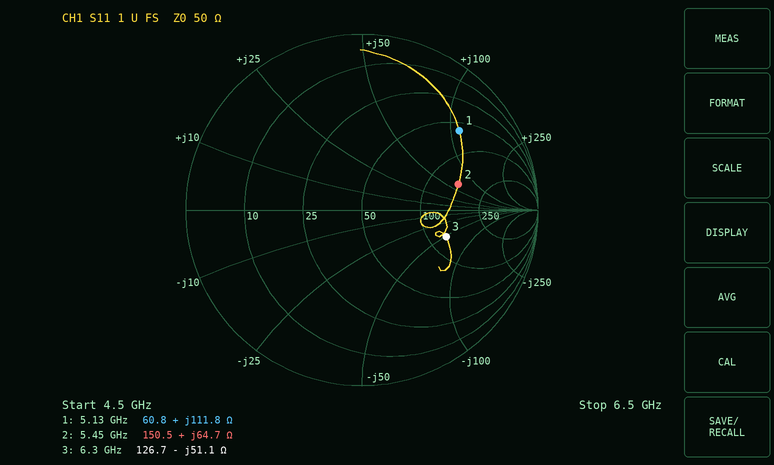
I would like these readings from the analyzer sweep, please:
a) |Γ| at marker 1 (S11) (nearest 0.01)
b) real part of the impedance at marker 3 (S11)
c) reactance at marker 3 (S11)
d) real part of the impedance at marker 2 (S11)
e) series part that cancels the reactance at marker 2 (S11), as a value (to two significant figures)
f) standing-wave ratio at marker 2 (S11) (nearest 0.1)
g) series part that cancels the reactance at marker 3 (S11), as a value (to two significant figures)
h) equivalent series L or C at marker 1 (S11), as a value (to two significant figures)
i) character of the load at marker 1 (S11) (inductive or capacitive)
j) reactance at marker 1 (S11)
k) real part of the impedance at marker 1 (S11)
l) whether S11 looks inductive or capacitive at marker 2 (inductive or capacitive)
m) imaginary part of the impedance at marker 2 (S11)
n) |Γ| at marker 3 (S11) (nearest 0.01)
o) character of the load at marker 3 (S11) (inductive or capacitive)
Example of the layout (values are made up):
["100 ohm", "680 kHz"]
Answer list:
["0.71", "126.7 Ω", "-51.1 Ω", "150.5 Ω", "450 fF", "3.6", "1.3 nH", "3.5 nH", "inductive", "+111.8 Ω", "60.8 Ω", "inductive", "+64.7 Ω", "0.50", "capacitive"]
